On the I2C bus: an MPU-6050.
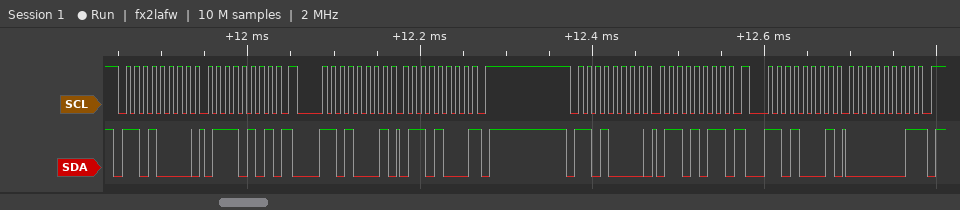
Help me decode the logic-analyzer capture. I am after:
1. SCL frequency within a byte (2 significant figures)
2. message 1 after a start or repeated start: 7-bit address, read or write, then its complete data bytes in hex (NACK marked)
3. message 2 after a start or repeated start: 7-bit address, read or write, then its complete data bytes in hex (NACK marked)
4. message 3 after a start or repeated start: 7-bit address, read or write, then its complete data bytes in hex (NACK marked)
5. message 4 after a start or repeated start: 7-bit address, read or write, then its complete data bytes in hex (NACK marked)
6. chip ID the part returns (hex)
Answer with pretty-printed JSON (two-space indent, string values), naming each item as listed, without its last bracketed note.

{
  "SCL frequency within a byte": "100 kHz",
  "message 1 after a start or repeated start: 7-bit address, read or write, then its complete data bytes in hex": "0x68 write: 75",
  "message 2 after a start or repeated start: 7-bit address, read or write, then its complete data bytes in hex": "0x68 read: 68 NACK",
  "message 3 after a start or repeated start: 7-bit address, read or write, then its complete data bytes in hex": "0x68 write: 6B",
  "message 4 after a start or repeated start: 7-bit address, read or write, then its complete data bytes in hex": "0x68 read: 01 NACK",
  "chip ID the part returns": "0x68"
}
